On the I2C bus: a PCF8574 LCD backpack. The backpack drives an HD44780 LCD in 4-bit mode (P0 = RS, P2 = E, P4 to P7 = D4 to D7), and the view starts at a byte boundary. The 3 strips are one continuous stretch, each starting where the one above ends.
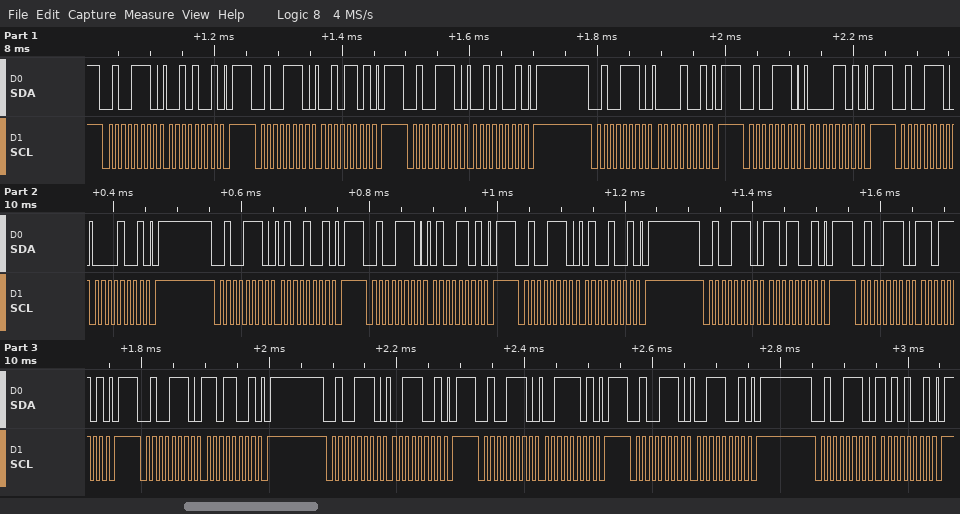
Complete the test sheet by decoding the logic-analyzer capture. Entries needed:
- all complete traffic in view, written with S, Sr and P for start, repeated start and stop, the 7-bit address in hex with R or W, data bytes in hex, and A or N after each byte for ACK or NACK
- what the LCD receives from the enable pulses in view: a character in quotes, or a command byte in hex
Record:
S 27W A 29 A P S 27W A 2D A P S 27W A 29 A P S 27W A 09 A P S 27W A 0D A P S 27W A 09 A P S 27W A 49 A P S 27W A 4D A P S 27W A 49 A P S 27W A D9 A P S 27W A DD A P S 27W A D9 A P S 27W A 39 A P S 27W A 3D A P S 27W A 39 A P S 27W A A9 A P
' ' 'M'
